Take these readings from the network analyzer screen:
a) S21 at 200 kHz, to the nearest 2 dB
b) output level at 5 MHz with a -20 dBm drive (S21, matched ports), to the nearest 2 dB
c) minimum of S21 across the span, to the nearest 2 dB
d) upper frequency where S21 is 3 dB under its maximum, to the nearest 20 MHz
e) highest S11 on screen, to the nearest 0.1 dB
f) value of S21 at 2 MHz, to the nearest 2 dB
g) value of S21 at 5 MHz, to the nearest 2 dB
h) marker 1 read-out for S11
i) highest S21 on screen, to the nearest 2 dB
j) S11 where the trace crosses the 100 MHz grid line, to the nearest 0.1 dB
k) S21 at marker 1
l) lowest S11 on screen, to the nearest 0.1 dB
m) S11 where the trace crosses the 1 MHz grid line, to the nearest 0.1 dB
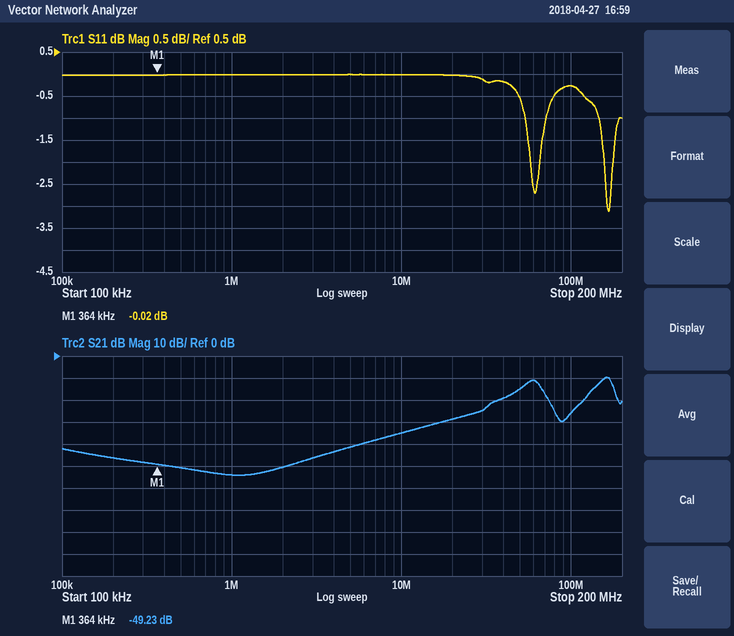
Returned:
-46 dB
-62 dBm
-54 dB
180 MHz
0.0 dB
-50 dB
-42 dB
-0.02 dB
-10 dB
-0.3 dB
-49.23 dB
-3.1 dB
0.0 dB
